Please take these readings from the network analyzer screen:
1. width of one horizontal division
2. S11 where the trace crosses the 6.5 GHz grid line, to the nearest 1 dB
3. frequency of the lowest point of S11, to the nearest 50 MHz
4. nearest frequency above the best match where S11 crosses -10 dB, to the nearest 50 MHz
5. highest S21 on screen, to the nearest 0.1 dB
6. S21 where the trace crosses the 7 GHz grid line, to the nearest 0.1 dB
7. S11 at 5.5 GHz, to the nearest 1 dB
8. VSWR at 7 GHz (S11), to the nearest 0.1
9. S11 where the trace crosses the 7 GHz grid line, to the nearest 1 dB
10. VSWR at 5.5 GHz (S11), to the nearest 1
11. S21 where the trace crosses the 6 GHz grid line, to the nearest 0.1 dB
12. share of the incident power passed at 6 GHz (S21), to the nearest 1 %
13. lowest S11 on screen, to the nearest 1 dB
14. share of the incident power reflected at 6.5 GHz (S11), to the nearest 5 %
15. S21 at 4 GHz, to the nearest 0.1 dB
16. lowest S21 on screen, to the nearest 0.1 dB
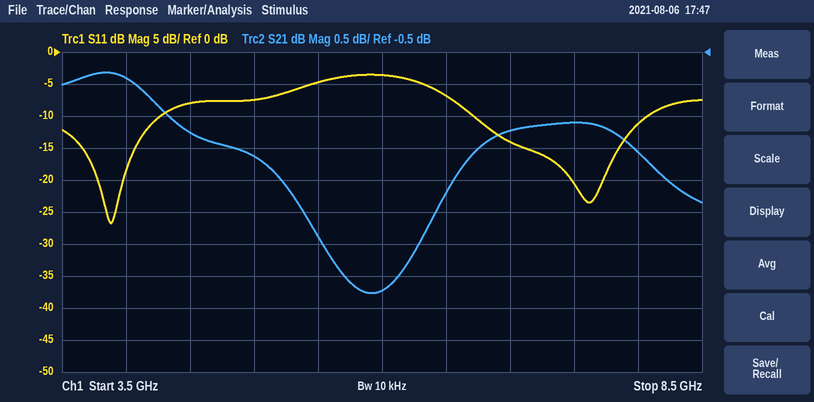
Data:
500 MHz
-7 dB
3.90 GHz
4.25 GHz
-0.8 dB
-1.7 dB
-5 dB
1.5
-14 dB
4
-4.2 dB
38 %
-27 dB
20 %
-0.9 dB
-4.3 dB
